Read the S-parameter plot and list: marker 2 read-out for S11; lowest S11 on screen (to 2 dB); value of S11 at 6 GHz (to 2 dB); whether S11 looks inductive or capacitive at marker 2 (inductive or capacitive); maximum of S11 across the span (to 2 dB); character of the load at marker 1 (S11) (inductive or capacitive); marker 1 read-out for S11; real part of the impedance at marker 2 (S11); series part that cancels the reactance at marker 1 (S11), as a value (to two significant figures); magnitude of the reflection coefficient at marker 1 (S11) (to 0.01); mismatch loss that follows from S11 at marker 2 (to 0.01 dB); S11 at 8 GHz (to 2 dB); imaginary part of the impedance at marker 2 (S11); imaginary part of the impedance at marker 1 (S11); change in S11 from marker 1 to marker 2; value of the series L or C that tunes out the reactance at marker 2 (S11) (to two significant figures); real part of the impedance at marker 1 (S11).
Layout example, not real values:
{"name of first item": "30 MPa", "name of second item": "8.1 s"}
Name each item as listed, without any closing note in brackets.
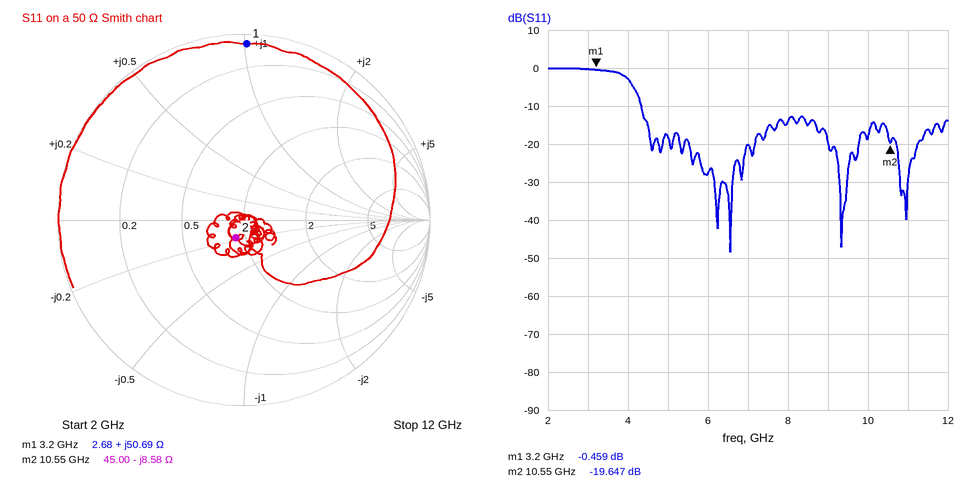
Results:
{"marker 2 read-out for S11": "-19.647 dB", "lowest S11 on screen": "-48 dB", "value of S11 at 6 GHz": "-28 dB", "whether S11 looks inductive or capacitive at marker 2": "capacitive", "maximum of S11 across the span": "0 dB", "character of the load at marker 1 (S11)": "inductive", "marker 1 read-out for S11": "-0.459 dB", "real part of the impedance at marker 2": "45.00 Ω", "series part that cancels the reactance at marker 1 (S11), as a value": "980 fF", "magnitude of the reflection coefficient at marker 1 (S11)": "0.95", "mismatch loss that follows from S11 at marker 2": "0.05 dB", "S11 at 8 GHz": "-14 dB", "imaginary part of the impedance at marker 2": "-8.58 Ω", "imaginary part of the impedance at marker 1": "+50.69 Ω", "change in S11 from marker 1 to marker 2": "-19.188 dB", "value of the series L or C that tunes out the reactance at marker 2 (S11)": "130 pH", "real part of the impedance at marker 1": "2.68 Ω"}
